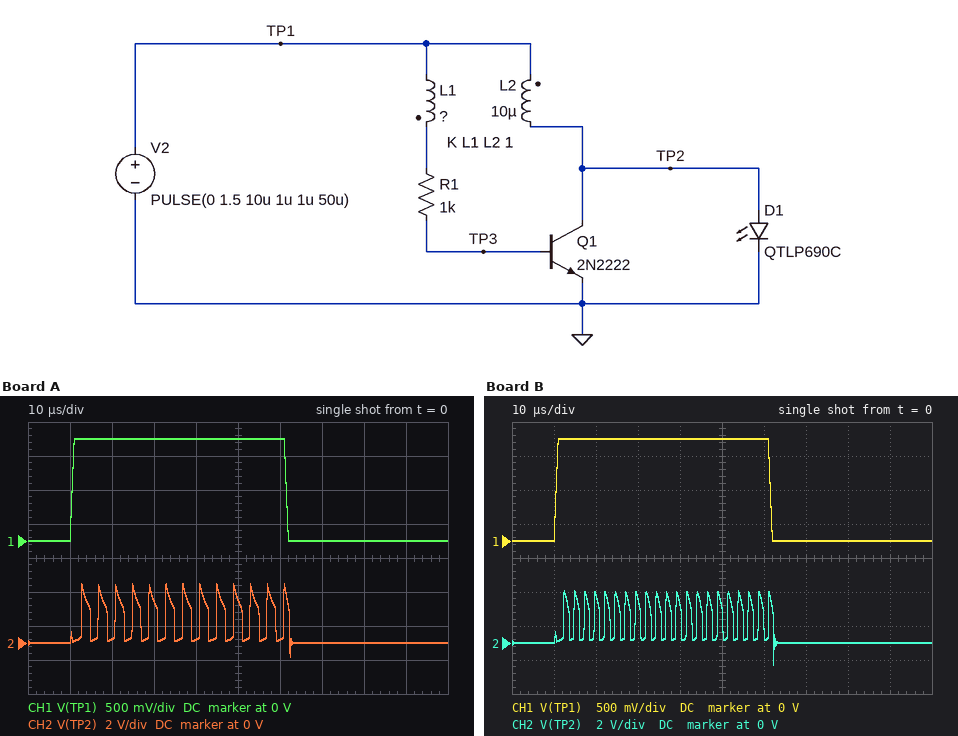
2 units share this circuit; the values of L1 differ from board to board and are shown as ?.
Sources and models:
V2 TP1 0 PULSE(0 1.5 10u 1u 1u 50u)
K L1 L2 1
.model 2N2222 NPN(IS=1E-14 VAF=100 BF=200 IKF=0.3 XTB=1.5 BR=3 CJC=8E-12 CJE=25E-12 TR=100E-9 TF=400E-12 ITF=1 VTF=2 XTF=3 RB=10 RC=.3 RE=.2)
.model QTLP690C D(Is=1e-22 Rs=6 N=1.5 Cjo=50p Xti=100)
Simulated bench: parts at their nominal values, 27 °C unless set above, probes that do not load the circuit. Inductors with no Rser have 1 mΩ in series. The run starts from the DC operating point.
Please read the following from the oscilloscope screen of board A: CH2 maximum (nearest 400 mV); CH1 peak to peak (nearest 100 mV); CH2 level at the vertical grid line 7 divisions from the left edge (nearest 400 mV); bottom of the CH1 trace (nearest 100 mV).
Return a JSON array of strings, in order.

["3.6 V", "1.5 V", "0 V", "0 V"]
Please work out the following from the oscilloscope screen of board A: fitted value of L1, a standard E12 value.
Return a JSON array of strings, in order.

["18 µH"]
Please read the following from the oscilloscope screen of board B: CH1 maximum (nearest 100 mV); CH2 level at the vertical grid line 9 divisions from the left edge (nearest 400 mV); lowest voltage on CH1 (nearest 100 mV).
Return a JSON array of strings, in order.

["1.5 V", "0 V", "0 V"]
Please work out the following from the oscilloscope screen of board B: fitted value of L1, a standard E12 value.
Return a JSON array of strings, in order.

["4.7 µH"]
